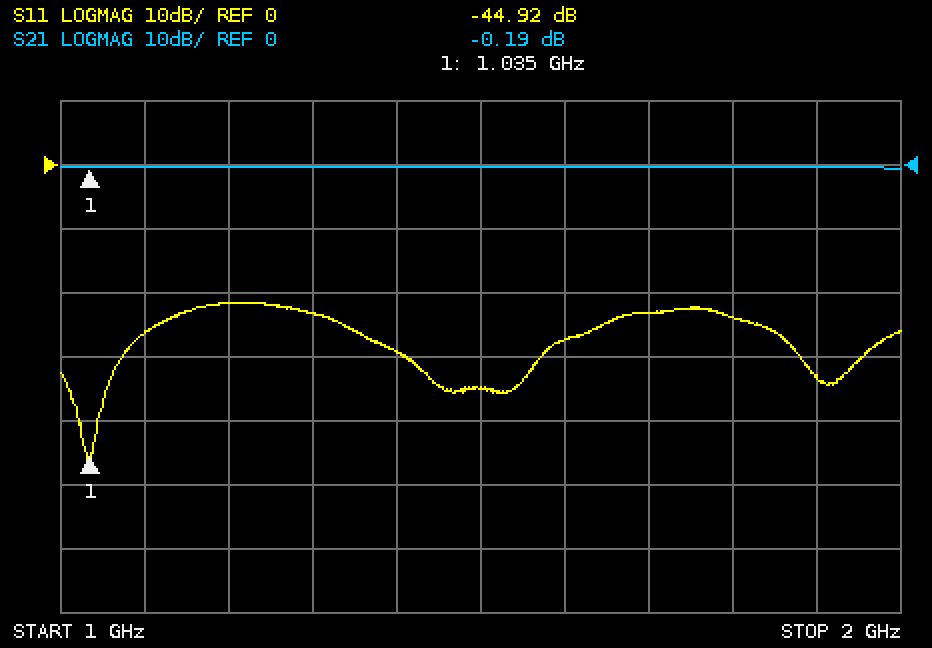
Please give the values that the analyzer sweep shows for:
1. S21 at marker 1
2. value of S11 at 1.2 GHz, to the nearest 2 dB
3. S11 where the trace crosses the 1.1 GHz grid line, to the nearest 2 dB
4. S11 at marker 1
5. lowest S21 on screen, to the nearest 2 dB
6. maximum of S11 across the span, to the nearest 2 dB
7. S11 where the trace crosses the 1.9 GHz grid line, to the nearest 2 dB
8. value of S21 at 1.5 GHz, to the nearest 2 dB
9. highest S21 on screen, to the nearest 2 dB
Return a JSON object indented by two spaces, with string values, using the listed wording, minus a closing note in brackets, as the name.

{
  "S21 at marker 1": "-0.19 dB",
  "value of S11 at 1.2 GHz, to the nearest 2 dB": "-22 dB",
  "S11 where the trace crosses the 1.1 GHz grid line, to the nearest 2 dB": "-26 dB",
  "S11 at marker 1": "-44.92 dB",
  "lowest S21 on screen, to the nearest 2 dB": "0 dB",
  "maximum of S11 across the span, to the nearest 2 dB": "-22 dB",
  "S11 where the trace crosses the 1.9 GHz grid line, to the nearest 2 dB": "-34 dB",
  "value of S21 at 1.5 GHz, to the nearest 2 dB": "0 dB",
  "highest S21 on screen, to the nearest 2 dB": "0 dB"
}
